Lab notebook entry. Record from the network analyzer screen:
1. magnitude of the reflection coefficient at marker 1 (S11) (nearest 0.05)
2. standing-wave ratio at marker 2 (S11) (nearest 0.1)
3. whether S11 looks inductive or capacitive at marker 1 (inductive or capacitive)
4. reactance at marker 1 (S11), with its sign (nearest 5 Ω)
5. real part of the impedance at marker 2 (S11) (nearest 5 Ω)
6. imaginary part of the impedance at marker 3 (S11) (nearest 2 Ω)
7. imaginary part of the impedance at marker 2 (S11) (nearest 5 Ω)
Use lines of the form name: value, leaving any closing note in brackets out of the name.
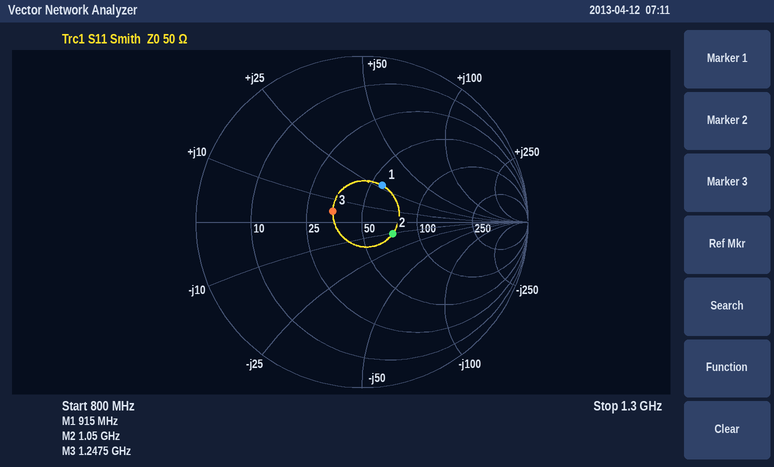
magnitude of the reflection coefficient at marker 1 (S11): 0.25
standing-wave ratio at marker 2 (S11): 1.5
whether S11 looks inductive or capacitive at marker 1: inductive
reactance at marker 1 (S11), with its sign: +25 Ω
real part of the impedance at marker 2 (S11): 70 Ω
imaginary part of the impedance at marker 3 (S11): +4 Ω
imaginary part of the impedance at marker 2 (S11): -10 Ω
